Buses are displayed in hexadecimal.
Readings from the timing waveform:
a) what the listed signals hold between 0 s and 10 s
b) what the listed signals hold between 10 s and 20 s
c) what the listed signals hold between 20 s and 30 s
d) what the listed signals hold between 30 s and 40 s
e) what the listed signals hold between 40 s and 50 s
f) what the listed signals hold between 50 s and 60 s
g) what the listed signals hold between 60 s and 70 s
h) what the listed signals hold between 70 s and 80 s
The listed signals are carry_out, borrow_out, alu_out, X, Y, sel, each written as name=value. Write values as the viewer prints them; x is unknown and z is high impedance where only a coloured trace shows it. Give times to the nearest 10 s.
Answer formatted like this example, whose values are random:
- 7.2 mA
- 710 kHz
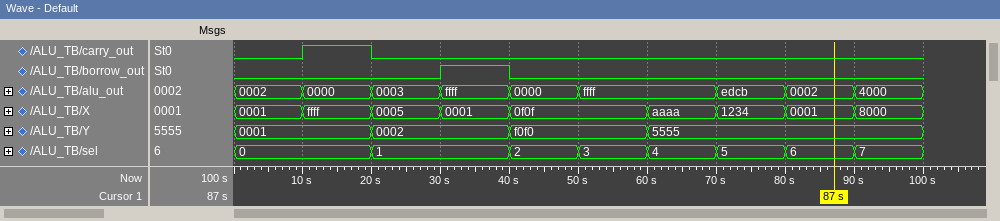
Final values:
- carry_out=0, borrow_out=0, alu_out=0002, X=0001, Y=0001, sel=0
- carry_out=1, borrow_out=0, alu_out=0000, X=ffff, Y=0001, sel=0
- carry_out=0, borrow_out=0, alu_out=0003, X=0005, Y=0002, sel=1
- carry_out=0, borrow_out=1, alu_out=ffff, X=0001, Y=0002, sel=1
- carry_out=0, borrow_out=0, alu_out=0000, X=0f0f, Y=f0f0, sel=2
- carry_out=0, borrow_out=0, alu_out=ffff, X=0f0f, Y=f0f0, sel=3
- carry_out=0, borrow_out=0, alu_out=ffff, X=aaaa, Y=5555, sel=4
- carry_out=0, borrow_out=0, alu_out=edcb, X=1234, Y=5555, sel=5
